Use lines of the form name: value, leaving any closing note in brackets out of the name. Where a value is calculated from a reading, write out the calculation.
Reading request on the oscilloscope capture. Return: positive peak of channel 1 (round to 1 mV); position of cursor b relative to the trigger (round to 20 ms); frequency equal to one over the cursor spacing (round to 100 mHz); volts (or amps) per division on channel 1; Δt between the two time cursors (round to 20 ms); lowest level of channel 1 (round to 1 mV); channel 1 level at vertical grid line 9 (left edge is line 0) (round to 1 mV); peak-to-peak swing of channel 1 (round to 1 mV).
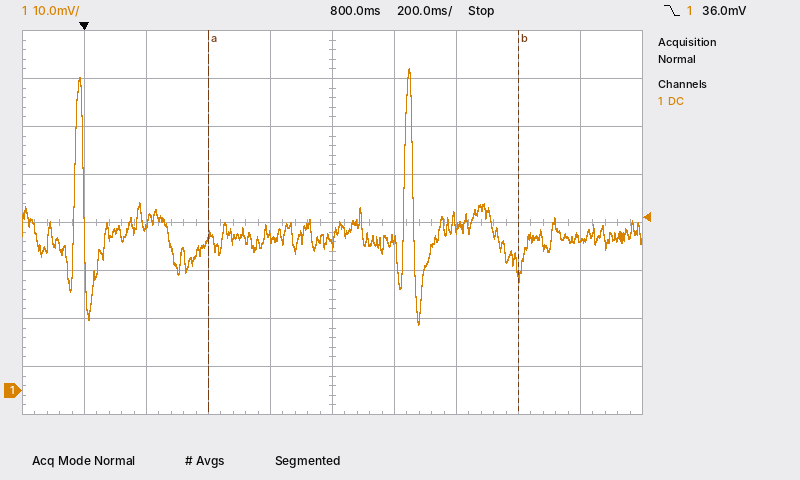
positive peak of channel 1: 67 mV
position of cursor b relative to the trigger: +1.40 s
frequency equal to one over the cursor spacing: 1 / 1.00 s ≈ 1.0 Hz
volts (or amps) per division on channel 1: 10 mV
Δt between the two time cursors: 1.00 s
lowest level of channel 1: 14 mV
channel 1 level at vertical grid line 9 (left edge is line 0): 32 mV
peak-to-peak swing of channel 1: 67 mV − (14 mV) = 53 mV
